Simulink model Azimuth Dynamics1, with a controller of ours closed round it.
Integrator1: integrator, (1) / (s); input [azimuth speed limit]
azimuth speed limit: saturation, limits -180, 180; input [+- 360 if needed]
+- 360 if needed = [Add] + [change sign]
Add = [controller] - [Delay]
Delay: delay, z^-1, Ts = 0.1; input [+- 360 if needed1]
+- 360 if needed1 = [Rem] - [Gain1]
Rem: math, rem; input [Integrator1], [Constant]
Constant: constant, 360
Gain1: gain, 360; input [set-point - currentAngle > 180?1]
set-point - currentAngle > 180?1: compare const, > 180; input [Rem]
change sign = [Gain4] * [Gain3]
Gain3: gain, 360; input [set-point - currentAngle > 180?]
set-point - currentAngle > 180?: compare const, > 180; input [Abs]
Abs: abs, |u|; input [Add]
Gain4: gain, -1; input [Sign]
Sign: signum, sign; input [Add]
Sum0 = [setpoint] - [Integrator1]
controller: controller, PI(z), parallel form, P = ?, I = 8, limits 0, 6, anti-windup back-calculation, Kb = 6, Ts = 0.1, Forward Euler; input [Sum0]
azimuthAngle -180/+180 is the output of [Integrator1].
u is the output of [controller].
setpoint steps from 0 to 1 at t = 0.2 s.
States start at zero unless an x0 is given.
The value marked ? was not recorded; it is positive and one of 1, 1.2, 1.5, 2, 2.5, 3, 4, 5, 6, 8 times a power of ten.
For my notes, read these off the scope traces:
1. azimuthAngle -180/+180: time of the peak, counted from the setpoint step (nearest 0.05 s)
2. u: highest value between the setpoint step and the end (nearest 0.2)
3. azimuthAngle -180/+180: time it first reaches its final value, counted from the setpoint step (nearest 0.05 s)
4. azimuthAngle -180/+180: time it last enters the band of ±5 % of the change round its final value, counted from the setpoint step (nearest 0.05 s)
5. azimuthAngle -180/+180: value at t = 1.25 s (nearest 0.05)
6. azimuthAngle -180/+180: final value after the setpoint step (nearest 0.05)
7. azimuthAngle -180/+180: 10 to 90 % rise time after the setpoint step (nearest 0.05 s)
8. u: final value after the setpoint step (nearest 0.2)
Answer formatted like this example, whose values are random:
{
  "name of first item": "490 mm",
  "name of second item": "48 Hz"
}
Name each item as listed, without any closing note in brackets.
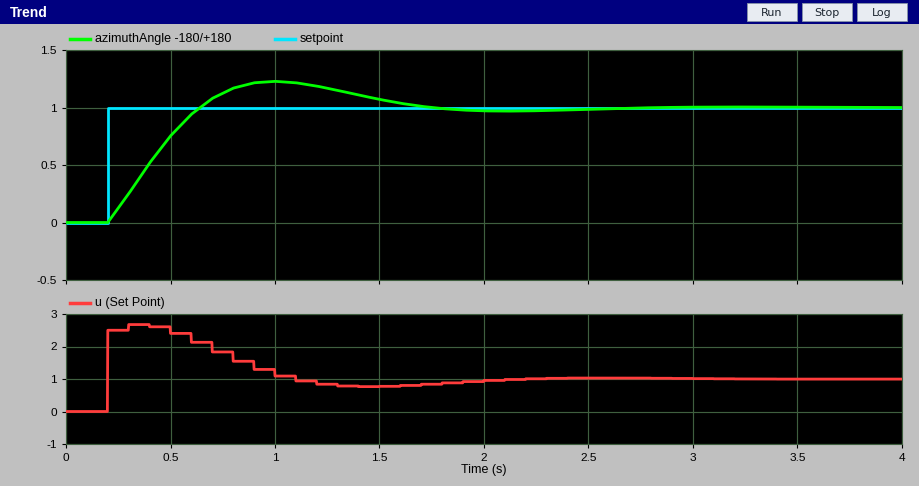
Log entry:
{
  "azimuthAngle -180/+180: time of the peak, counted from the setpoint step": "0.80 s",
  "u: highest value between the setpoint step and the end": "2.6",
  "azimuthAngle -180/+180: time it first reaches its final value, counted from the setpoint step": "0.45 s",
  "azimuthAngle -180/+180: time it last enters the band of ±5 % of the change round its final value, counted from the setpoint step": "1.35 s",
  "azimuthAngle -180/+180: value at t = 1.25 s": "1.15",
  "azimuthAngle -180/+180: final value after the setpoint step": "1.00",
  "azimuthAngle -180/+180: 10 to 90 % rise time after the setpoint step": "0.35 s",
  "u: final value after the setpoint step": "1.0"
}
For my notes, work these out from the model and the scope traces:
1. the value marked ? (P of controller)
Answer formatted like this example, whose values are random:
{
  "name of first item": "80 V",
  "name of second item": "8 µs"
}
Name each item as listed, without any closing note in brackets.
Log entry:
{
  "the value marked ?": "2.5"
}
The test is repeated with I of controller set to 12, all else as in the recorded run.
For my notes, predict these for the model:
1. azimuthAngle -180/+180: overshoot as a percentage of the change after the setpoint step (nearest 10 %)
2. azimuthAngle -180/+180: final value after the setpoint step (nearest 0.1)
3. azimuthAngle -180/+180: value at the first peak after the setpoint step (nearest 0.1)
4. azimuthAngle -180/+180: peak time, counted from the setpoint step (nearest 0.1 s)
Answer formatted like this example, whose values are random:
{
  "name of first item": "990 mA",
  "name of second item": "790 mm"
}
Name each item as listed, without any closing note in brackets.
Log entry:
{
  "azimuthAngle -180/+180: overshoot as a percentage of the change after the setpoint step": "40 %",
  "azimuthAngle -180/+180: final value after the setpoint step": "1.0",
  "azimuthAngle -180/+180: value at the first peak after the setpoint step": "1.4",
  "azimuthAngle -180/+180: peak time, counted from the setpoint step": "0.7 s"
}
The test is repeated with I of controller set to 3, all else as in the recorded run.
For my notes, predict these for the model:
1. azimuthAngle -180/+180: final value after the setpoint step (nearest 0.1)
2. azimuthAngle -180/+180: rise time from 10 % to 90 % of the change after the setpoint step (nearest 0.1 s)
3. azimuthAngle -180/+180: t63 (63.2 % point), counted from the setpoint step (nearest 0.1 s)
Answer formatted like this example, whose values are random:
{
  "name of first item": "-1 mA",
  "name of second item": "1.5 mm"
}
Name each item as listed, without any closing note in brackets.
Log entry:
{
  "azimuthAngle -180/+180: final value after the setpoint step": "1.0",
  "azimuthAngle -180/+180: rise time from 10 % to 90 % of the change after the setpoint step": "0.6 s",
  "azimuthAngle -180/+180: t63 (63.2 % point), counted from the setpoint step": "0.3 s"
}
